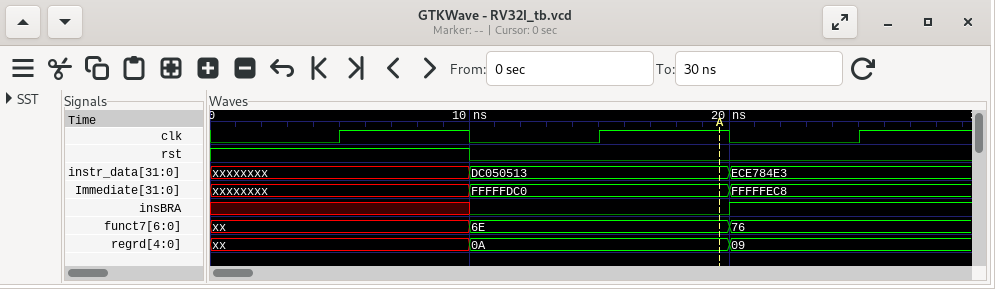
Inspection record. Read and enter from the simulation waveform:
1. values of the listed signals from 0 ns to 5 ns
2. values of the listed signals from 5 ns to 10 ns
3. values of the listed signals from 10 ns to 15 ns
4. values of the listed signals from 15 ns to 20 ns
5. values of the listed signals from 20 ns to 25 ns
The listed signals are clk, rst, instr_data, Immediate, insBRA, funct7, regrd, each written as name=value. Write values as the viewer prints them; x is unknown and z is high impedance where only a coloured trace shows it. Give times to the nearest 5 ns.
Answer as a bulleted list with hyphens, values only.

- clk=0, rst=1, instr_data=xxxxxxxx, Immediate=xxxxxxxx, insBRA=x, funct7=xx, regrd=xx
- clk=1, rst=1, instr_data=xxxxxxxx, Immediate=xxxxxxxx, insBRA=x, funct7=xx, regrd=xx
- clk=0, rst=0, instr_data=DC050513, Immediate=FFFFFDC0, insBRA=0, funct7=6E, regrd=0A
- clk=1, rst=0, instr_data=DC050513, Immediate=FFFFFDC0, insBRA=0, funct7=6E, regrd=0A
- clk=0, rst=0, instr_data=ECE784E3, Immediate=FFFFFEC8, insBRA=1, funct7=76, regrd=09
